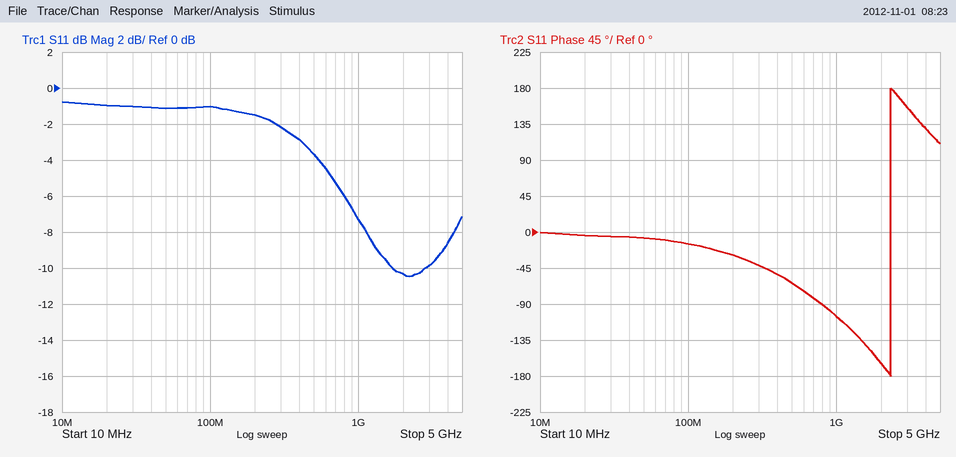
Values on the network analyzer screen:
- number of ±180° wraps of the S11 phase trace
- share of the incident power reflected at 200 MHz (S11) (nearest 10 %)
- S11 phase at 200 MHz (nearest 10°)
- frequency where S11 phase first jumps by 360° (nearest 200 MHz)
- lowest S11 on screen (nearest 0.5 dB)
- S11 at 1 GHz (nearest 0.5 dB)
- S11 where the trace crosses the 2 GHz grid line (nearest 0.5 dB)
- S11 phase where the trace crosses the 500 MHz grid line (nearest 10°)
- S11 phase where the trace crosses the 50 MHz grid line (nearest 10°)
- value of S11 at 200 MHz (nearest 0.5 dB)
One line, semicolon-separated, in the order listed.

1; 70 %; -30°; 2.4 GHz; -10.5 dB; -7.5 dB; -10.5 dB; -60°; -10°; -1.5 dB
